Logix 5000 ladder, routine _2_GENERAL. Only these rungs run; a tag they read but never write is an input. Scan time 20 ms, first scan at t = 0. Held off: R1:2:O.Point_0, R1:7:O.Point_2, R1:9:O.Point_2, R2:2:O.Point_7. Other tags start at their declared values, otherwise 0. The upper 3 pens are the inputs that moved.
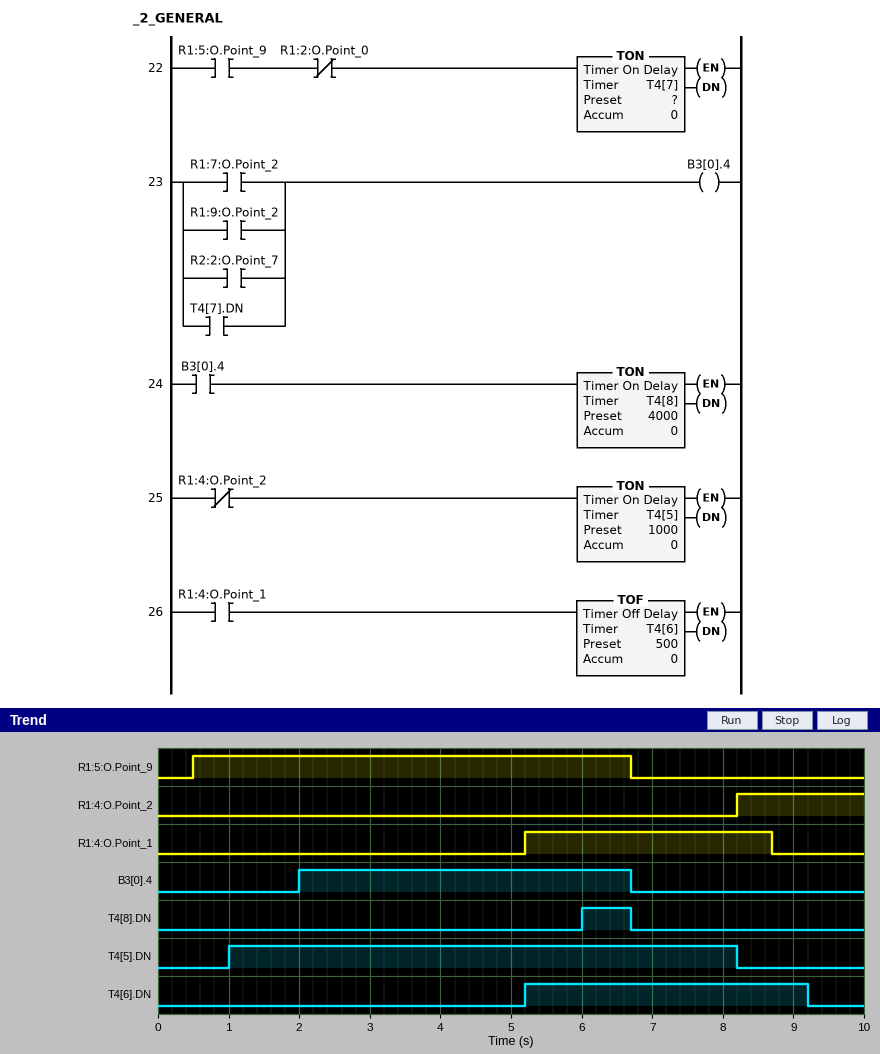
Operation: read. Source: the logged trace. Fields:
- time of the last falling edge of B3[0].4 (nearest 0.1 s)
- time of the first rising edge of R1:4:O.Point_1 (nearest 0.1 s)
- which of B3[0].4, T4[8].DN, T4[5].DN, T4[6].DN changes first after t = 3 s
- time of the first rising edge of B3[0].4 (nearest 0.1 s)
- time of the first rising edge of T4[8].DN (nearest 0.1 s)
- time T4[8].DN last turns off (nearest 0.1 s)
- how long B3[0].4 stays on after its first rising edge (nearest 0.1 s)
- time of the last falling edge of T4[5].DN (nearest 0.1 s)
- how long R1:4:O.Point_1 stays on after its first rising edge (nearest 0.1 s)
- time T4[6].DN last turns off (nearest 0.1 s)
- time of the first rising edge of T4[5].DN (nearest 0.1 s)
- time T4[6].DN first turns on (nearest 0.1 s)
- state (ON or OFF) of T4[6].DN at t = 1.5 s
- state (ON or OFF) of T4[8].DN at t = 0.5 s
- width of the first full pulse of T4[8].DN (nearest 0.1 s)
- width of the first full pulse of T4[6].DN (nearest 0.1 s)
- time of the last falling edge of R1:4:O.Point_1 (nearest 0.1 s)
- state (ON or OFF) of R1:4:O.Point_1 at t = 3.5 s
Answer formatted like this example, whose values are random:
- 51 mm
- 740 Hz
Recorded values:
- 6.7 s
- 5.2 s
- T4[6].DN
- 2.0 s
- 6.0 s
- 6.7 s
- 4.7 s
- 8.2 s
- 3.5 s
- 9.2 s
- 1.0 s
- 5.2 s
- OFF
- OFF
- 0.7 s
- 4.0 s
- 8.7 s
- OFF
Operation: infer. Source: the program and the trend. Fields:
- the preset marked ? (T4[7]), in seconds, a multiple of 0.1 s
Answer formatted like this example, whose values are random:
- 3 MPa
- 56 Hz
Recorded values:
- 1.5 s
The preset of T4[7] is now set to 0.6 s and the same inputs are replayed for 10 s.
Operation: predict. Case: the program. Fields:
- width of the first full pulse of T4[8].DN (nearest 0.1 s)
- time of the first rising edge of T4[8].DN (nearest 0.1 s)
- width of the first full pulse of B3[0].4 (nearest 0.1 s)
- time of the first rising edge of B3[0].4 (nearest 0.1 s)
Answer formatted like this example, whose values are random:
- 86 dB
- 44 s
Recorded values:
- 1.6 s
- 5.1 s
- 5.6 s
- 1.1 s
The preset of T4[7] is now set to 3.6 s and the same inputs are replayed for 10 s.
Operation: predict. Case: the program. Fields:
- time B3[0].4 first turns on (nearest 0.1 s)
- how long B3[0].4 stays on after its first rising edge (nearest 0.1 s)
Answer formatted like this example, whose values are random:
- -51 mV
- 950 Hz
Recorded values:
- 4.1 s
- 2.6 s
